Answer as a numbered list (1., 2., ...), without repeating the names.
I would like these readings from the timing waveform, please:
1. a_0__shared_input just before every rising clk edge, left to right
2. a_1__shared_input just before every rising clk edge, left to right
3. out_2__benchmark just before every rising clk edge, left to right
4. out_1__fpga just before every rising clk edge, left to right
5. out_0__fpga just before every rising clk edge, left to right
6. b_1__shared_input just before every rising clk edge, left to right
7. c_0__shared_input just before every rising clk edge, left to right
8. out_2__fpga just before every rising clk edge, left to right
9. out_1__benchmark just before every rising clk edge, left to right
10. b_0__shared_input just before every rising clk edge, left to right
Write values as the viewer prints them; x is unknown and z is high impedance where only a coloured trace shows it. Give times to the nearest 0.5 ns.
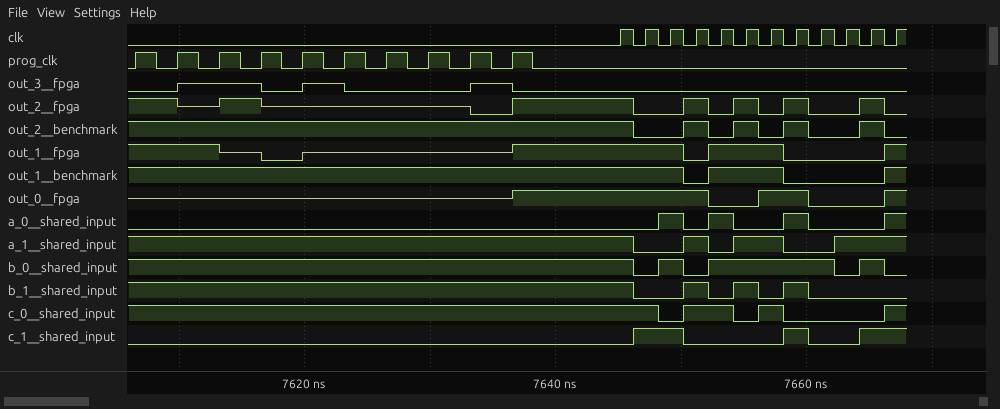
1. 0 0 1 0 1 0 0 1 0 0 0 1
2. 1 0 0 1 0 1 1 0 0 1 1 1
3. 1 0 0 1 0 1 0 1 0 0 1 0
4. 1 1 1 0 1 1 1 0 0 0 0 1
5. 1 1 1 1 0 0 1 1 0 0 0 1
6. 1 0 0 1 0 1 0 1 0 0 0 0
7. 1 1 0 1 1 0 1 0 0 0 0 1
8. 1 0 0 1 0 1 0 1 0 0 1 0
9. 1 1 1 0 1 1 1 0 0 0 0 1
10. 1 0 1 0 1 1 1 1 1 0 1 0
